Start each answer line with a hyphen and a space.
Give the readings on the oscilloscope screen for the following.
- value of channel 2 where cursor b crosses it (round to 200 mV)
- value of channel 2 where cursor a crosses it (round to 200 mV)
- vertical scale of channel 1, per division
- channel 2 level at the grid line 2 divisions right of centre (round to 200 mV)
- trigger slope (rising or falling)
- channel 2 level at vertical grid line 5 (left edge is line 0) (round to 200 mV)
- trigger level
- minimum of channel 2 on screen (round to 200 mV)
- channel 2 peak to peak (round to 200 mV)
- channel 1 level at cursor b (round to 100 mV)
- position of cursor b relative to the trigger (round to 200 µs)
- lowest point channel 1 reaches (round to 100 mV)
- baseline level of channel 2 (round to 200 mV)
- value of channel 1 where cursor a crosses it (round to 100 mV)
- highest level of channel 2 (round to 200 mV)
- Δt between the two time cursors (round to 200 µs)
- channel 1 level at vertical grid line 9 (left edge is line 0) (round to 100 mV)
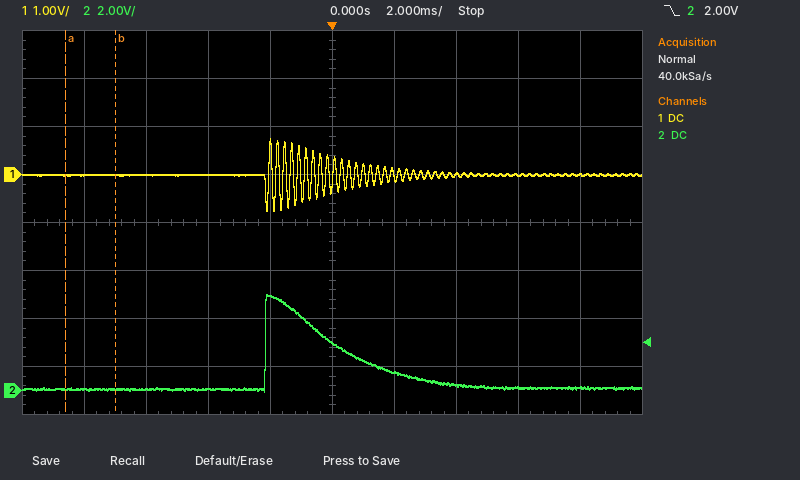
- 0.0 V
- 0.0 V
- 1 V
- 200 mV
- falling
- 2.0 V
- 2.00 V
- 0.0 V
- 4.0 V
- 0.0 V
- -7.0 ms
- -800 mV
- 0.0 V
- 0.0 V
- 4.0 V
- 1.6 ms
- 0.0 V
